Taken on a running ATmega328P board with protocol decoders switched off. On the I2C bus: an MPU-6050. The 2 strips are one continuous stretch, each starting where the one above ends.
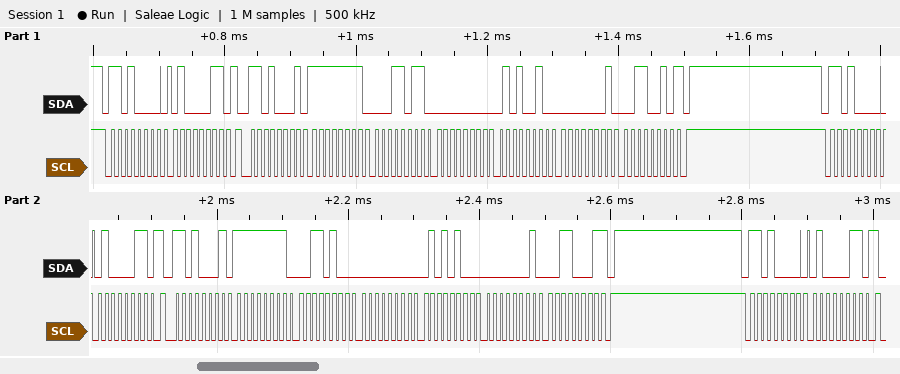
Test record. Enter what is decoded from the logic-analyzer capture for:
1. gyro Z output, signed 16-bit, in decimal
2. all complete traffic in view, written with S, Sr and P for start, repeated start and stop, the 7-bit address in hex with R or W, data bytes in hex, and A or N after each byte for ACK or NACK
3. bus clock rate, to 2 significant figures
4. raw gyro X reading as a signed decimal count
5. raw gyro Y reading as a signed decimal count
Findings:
306
S 68W A 43 A Sr 68R A FF A 1B A 00 A 52 A 01 A 32 N P S 68W A 43 A Sr 68R A FF A 34 A 00 A 54 A 01 A 31 N P S 68W A 43 A
100 kHz
-229
82
